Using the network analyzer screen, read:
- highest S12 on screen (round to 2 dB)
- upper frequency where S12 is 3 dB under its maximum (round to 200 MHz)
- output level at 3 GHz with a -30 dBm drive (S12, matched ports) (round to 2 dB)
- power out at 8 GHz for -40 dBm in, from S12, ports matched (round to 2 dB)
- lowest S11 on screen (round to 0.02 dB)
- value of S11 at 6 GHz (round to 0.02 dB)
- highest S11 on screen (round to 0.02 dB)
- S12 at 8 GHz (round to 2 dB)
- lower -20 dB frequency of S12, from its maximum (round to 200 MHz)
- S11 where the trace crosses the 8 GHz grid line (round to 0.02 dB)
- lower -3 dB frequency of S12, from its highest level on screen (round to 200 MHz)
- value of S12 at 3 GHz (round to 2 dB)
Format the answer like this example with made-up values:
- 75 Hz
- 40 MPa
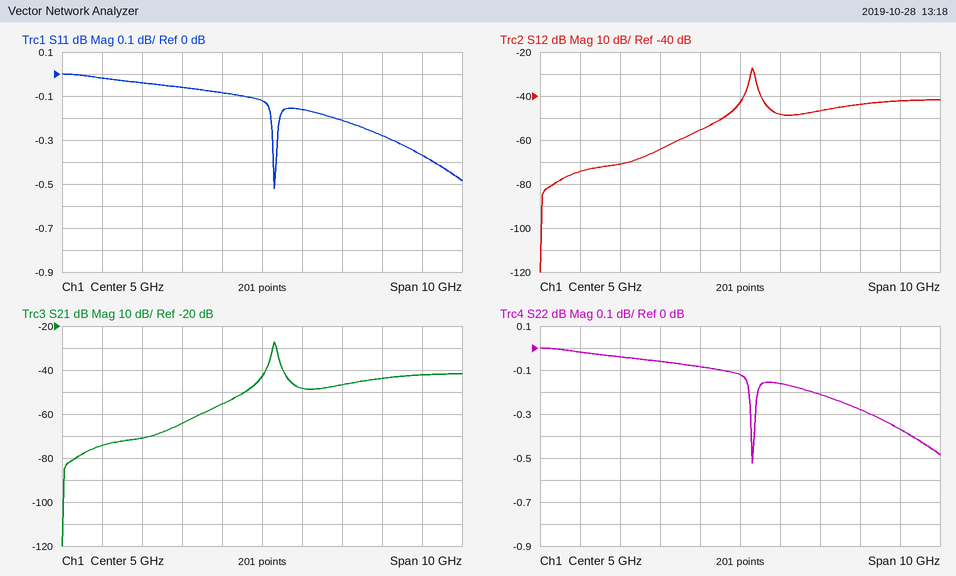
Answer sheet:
- -28 dB
- 5.4 GHz
- -94 dBm
- -84 dBm
- -0.52 dB
- -0.16 dB
- 0.00 dB
- -44 dB
- 4.8 GHz
- -0.28 dB
- 5.2 GHz
- -64 dB
